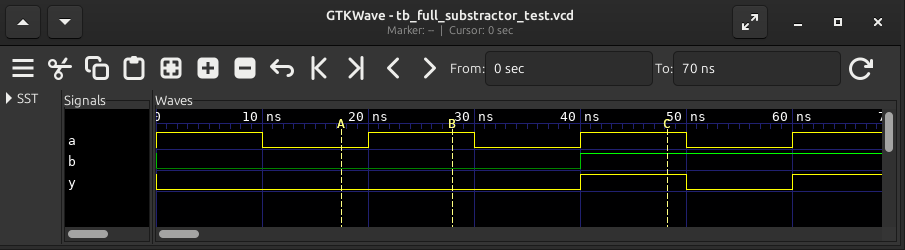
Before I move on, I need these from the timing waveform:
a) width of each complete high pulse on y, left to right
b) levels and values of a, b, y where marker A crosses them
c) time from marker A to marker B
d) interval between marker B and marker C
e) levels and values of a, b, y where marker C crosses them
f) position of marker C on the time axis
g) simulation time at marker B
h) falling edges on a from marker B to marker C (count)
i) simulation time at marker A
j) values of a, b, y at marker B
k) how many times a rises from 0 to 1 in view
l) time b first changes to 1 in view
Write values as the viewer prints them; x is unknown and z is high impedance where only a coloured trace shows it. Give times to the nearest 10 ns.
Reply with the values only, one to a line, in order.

10 ns
a=0, b=0, y=0
10 ns
20 ns
a=1, b=1, y=1
50 ns
30 ns
1
20 ns
a=1, b=0, y=0
3
40 ns
